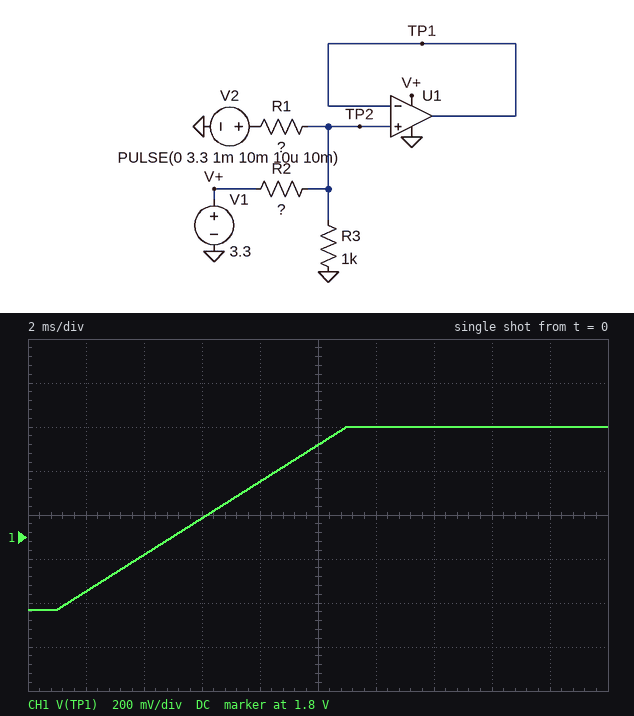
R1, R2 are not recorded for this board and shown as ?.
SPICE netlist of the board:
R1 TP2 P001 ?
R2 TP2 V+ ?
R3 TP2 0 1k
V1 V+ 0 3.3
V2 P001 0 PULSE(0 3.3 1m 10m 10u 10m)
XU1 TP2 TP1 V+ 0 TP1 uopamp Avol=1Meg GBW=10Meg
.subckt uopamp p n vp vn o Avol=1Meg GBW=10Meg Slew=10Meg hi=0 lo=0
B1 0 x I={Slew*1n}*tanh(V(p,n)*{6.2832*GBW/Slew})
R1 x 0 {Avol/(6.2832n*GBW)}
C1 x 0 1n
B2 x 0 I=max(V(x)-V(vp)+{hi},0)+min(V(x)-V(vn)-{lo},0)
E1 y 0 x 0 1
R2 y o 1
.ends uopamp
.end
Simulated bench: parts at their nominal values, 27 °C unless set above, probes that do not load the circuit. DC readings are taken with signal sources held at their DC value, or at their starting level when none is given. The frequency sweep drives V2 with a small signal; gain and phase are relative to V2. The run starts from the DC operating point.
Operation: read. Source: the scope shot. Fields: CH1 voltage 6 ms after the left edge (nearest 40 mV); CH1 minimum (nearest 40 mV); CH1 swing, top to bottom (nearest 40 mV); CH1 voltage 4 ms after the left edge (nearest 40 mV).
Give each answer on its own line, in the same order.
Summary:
1.88 V
1.48 V
840 mV
1.72 V
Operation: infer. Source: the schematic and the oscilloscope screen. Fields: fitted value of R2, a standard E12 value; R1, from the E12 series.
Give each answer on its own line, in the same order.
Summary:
680 Ω
1.2 kΩ
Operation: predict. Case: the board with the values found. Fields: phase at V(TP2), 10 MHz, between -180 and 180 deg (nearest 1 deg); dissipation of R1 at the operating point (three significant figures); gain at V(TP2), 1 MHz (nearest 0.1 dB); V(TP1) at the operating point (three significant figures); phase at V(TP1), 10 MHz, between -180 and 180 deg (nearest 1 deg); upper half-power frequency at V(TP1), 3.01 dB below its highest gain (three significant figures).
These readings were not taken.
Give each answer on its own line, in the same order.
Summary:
0 deg
1.80 mW
-12.0 dB
1.47 V
-45 deg
10.0 MHz
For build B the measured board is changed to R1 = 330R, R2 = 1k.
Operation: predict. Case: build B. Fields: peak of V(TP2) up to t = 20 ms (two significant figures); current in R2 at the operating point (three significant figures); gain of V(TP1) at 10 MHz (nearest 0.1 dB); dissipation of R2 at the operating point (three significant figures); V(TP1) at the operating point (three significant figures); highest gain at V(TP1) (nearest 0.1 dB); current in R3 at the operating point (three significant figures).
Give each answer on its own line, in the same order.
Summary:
2.6 V
2.64 mA
-7.4 dB
6.99 mW
656 mV
-4.4 dB
656 µA
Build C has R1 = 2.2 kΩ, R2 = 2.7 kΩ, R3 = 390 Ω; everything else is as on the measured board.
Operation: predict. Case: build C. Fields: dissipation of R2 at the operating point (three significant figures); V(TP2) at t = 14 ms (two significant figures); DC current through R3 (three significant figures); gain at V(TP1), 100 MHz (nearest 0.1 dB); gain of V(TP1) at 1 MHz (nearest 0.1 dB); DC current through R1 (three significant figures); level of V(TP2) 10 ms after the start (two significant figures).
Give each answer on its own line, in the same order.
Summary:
3.20 mW
800 mV
925 µA
-37.5 dB
-17.5 dB
164 µA
760 mV
